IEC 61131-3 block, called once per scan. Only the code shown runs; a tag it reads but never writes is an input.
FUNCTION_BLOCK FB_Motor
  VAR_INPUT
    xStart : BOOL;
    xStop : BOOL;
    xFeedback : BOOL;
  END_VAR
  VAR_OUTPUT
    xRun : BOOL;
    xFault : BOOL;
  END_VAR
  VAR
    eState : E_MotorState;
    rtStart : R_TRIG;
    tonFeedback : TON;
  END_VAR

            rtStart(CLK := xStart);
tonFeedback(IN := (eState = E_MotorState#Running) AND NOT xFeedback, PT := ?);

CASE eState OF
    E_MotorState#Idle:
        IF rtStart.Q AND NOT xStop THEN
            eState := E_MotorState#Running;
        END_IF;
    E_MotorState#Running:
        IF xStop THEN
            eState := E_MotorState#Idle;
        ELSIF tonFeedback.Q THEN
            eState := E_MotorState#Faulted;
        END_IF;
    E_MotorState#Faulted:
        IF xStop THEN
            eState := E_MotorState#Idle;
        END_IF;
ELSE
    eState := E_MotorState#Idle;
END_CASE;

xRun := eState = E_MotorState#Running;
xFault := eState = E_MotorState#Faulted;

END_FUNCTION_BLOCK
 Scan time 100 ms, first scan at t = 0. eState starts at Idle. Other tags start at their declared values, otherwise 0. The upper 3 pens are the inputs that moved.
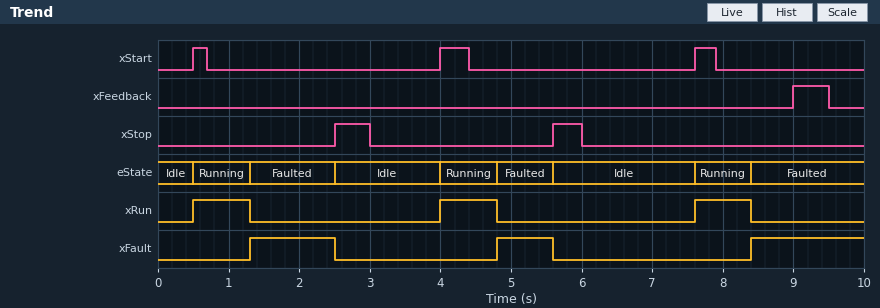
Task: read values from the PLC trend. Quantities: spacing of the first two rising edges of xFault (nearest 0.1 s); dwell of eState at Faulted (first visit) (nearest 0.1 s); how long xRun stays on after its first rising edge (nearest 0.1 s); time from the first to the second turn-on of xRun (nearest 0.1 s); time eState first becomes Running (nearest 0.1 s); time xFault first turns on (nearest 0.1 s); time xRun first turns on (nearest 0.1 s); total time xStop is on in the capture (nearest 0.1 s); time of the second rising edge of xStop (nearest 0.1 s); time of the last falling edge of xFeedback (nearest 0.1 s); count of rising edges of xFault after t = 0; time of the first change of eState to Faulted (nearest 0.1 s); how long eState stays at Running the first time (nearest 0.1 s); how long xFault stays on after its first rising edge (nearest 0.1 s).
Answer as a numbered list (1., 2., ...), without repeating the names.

1. 3.5 s
2. 1.2 s
3. 0.8 s
4. 3.5 s
5. 0.5 s
6. 1.3 s
7. 0.5 s
8. 0.9 s
9. 5.6 s
10. 9.5 s
11. 3
12. 1.3 s
13. 0.8 s
14. 1.2 s
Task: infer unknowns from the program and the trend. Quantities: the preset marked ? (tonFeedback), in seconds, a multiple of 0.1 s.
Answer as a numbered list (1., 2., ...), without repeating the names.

1. 0.7 s
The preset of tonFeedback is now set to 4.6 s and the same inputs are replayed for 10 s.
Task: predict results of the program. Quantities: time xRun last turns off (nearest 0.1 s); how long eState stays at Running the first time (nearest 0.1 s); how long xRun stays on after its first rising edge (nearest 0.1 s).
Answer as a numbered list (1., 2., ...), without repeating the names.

1. 5.6 s
2. 2.0 s
3. 2.0 s
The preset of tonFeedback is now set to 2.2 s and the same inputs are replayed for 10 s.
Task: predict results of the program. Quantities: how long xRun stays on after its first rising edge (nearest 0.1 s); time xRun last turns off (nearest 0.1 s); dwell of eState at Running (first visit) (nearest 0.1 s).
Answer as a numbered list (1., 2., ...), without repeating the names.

1. 2.0 s
2. 5.6 s
3. 2.0 s
